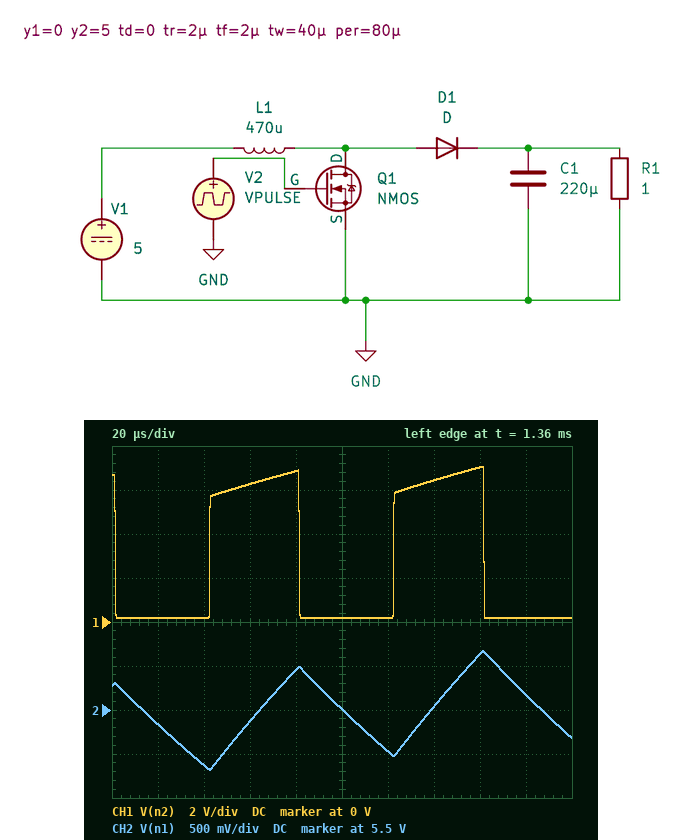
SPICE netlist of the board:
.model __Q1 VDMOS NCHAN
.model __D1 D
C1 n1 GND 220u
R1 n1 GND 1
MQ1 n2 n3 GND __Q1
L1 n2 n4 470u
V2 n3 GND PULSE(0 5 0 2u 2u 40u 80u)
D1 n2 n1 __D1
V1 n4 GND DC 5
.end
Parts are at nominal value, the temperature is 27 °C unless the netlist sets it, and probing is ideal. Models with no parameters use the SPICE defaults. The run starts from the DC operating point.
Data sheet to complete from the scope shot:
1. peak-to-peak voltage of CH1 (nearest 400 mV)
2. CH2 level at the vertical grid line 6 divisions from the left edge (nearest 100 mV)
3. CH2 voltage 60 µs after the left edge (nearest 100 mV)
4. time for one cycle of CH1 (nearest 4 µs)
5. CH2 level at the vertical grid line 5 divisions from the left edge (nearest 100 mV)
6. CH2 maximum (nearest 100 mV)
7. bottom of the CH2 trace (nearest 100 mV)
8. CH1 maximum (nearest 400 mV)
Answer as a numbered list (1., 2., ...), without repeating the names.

1. 6.8 V
2. 5.0 V
3. 5.4 V
4. 80 µs
5. 5.5 V
6. 6.2 V
7. 4.8 V
8. 7.2 V
